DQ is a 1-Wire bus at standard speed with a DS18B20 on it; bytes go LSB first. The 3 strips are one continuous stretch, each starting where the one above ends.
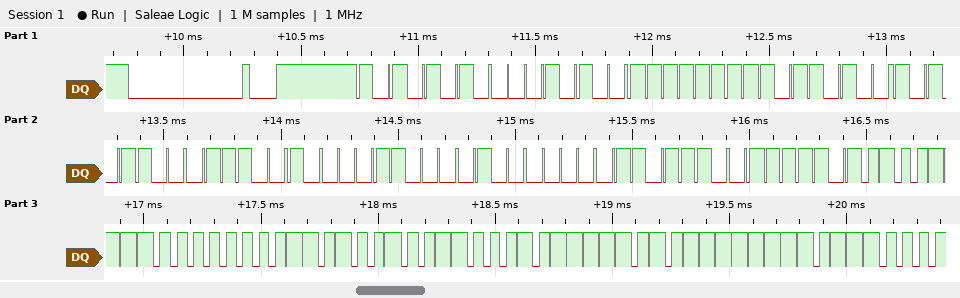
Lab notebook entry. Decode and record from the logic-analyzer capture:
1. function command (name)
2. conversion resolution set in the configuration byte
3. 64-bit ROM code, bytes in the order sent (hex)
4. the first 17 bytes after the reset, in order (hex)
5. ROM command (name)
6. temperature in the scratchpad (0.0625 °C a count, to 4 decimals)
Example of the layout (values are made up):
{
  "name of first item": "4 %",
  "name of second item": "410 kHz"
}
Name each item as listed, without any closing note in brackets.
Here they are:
{
  "function command": "Read Scratchpad",
  "conversion resolution set in the configuration byte": "11 bits",
  "64-bit ROM code, bytes in the order sent": "28 FF 2D 35 4E 18 02 76",
  "the first 17 bytes after the reset, in order": "55 28 FF 2D 35 4E 18 02 76 BE F2 00 4B 46 5F FF 0E",
  "ROM command": "Match ROM",
  "temperature in the scratchpad": "15.1250 °C"
}
